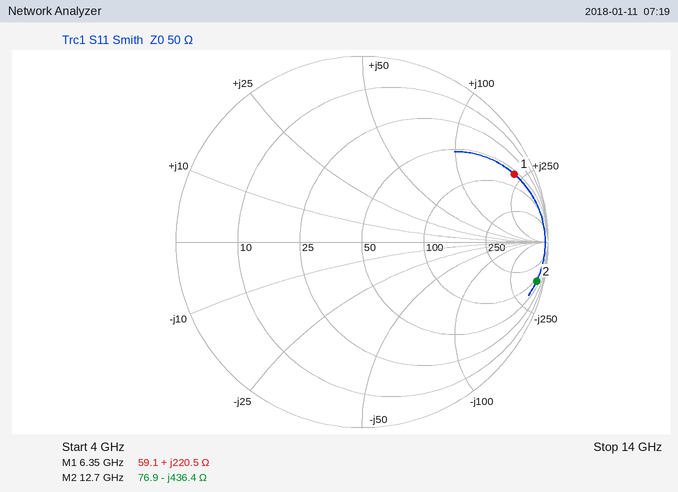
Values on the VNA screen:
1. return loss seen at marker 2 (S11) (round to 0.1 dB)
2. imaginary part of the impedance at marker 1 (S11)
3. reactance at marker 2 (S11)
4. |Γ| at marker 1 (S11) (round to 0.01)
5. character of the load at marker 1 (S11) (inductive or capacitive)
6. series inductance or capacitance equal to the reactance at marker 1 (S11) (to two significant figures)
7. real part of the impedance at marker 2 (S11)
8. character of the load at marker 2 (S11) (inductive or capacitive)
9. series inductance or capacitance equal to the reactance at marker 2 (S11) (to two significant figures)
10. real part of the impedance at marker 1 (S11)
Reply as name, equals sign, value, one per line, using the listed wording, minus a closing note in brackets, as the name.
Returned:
return loss seen at marker 2 (S11) = 0.3 dB
imaginary part of the impedance at marker 1 = +220.5 Ω
reactance at marker 2 = -436.4 Ω
|Γ| at marker 1 (S11) = 0.90
character of the load at marker 1 (S11) = inductive
series inductance or capacitance equal to the reactance at marker 1 (S11) = 5.5 nH
real part of the impedance at marker 2 = 76.9 Ω
character of the load at marker 2 (S11) = capacitive
series inductance or capacitance equal to the reactance at marker 2 (S11) = 29 fF
real part of the impedance at marker 1 = 59.1 Ω
